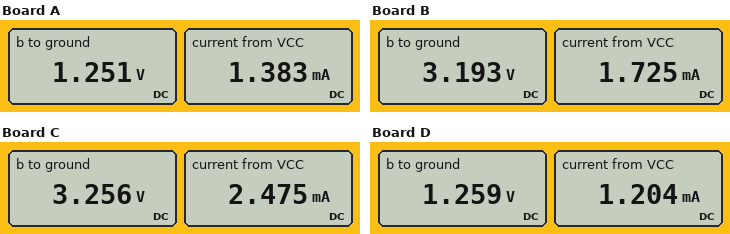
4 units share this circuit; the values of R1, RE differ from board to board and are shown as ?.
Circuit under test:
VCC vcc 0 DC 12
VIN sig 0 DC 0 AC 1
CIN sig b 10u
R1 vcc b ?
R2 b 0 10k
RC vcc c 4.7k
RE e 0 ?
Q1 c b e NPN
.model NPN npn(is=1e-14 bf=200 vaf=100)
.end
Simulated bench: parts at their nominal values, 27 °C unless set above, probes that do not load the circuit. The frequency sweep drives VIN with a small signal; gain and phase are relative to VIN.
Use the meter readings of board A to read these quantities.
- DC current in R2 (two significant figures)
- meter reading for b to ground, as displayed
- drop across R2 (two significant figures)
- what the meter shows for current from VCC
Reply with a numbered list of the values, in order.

1. 130 µA
2. 1.251 V
3. 1.3 V
4. 1.383 mA
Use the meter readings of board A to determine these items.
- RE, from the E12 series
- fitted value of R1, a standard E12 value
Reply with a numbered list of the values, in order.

1. 470 Ω
2. 82 kΩ
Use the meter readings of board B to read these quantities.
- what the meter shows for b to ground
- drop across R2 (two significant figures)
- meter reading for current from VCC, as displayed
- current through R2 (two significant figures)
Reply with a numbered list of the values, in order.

1. 3.193 V
2. 3.2 V
3. 1.725 mA
4. 320 µA
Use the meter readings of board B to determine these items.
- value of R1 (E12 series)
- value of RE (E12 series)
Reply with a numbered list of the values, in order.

1. 27 kΩ
2. 1.8 kΩ
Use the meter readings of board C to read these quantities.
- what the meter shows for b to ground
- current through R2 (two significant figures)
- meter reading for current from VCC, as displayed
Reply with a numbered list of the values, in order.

1. 3.256 V
2. 330 µA
3. 2.475 mA
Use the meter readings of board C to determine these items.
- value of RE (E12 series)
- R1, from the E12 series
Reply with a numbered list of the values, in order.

1. 1.2 kΩ
2. 18 kΩ
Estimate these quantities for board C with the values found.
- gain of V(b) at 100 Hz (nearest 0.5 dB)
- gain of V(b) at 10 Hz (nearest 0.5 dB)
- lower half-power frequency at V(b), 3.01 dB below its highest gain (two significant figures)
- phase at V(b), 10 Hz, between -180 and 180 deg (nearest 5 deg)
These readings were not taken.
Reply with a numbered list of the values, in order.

1. 0 dB
2. -6.5 dB
3. 18 Hz
4. 60 deg
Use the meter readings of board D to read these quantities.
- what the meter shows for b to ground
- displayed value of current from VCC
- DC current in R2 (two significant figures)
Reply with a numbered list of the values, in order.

1. 1.259 V
2. 1.204 mA
3. 130 µA
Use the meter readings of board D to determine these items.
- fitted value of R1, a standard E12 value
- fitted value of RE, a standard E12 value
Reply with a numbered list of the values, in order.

1. 82 kΩ
2. 560 Ω
